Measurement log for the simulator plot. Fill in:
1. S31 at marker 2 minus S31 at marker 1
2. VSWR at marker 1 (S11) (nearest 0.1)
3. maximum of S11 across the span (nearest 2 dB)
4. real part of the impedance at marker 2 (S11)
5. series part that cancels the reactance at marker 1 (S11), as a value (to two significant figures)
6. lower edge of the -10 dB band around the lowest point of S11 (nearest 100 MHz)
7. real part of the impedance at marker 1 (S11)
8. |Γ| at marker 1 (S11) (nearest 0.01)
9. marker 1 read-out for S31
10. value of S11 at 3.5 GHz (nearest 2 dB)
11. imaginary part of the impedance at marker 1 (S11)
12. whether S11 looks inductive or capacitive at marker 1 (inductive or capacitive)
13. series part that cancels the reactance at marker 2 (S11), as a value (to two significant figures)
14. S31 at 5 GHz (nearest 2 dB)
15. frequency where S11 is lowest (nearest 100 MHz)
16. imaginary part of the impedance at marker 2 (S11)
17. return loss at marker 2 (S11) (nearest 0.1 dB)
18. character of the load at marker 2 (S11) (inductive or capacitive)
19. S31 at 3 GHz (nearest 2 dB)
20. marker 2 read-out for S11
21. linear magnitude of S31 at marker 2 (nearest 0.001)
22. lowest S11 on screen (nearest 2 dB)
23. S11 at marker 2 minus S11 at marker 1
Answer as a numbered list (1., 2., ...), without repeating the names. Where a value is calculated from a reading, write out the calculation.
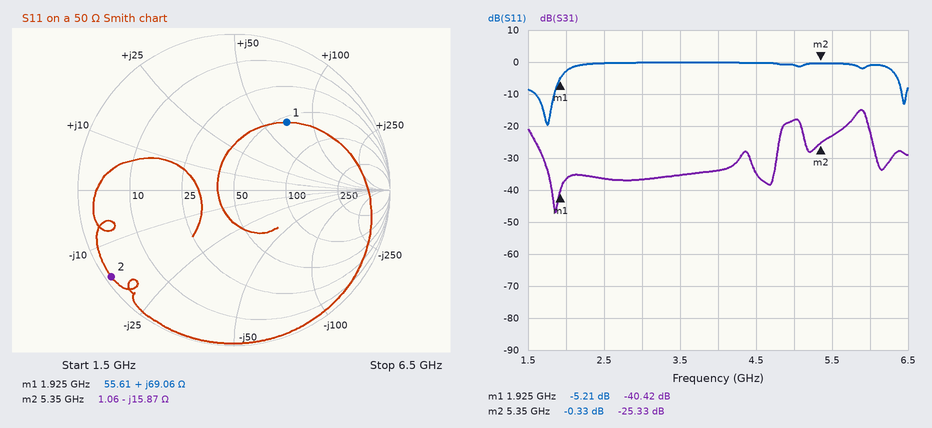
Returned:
1. -25.33 − (-40.42) = 15.09 dB
2. (1 + 0.5489)/(1 − 0.5489) ≈ 3.4
3. 0 dB
4. 1.06 Ω
5. C = 1/(2π × 1.925 GHz × 69.06 Ω) ≈ 1.2 pF
6. 1.6 GHz
7. 55.61 Ω
8. 0.55
9. -40.42 dB
10. 0 dB
11. +69.06 Ω
12. inductive
13. L = 15.87 Ω/(2π × 5.35 GHz) ≈ 472 pH, so 470 pH to two significant figures
14. -18 dB
15. 1.8 GHz
16. -15.87 Ω
17. 0.3 dB
18. capacitive
19. -36 dB
20. -0.33 dB
21. 10^(-25.33/20) ≈ 0.054
22. -20 dB
23. -0.33 − (-5.21) = 4.88 dB
